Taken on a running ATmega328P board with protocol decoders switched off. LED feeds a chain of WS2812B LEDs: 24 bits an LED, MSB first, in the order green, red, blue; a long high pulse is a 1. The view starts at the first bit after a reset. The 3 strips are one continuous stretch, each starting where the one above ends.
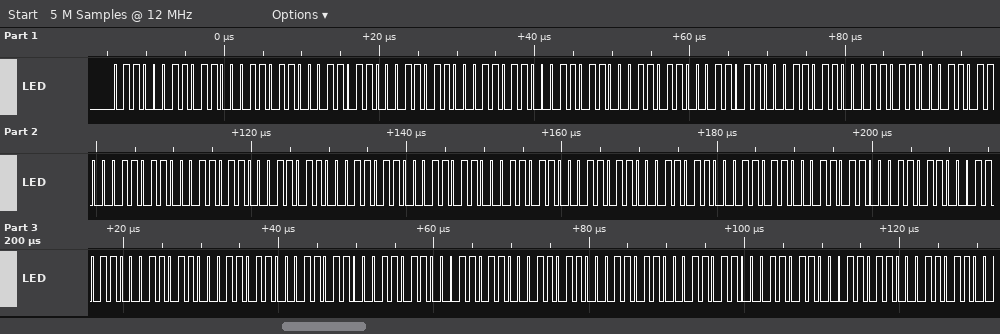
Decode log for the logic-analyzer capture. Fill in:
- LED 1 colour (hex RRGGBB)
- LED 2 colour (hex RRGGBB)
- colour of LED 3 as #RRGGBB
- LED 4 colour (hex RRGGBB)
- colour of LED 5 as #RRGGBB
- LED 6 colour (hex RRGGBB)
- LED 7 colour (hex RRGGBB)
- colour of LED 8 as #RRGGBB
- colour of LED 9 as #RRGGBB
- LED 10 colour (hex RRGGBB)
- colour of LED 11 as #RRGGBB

#636363
#636363
#636363
#636363
#636363
#636363
#636363
#636363
#636363
#636363
#636363
